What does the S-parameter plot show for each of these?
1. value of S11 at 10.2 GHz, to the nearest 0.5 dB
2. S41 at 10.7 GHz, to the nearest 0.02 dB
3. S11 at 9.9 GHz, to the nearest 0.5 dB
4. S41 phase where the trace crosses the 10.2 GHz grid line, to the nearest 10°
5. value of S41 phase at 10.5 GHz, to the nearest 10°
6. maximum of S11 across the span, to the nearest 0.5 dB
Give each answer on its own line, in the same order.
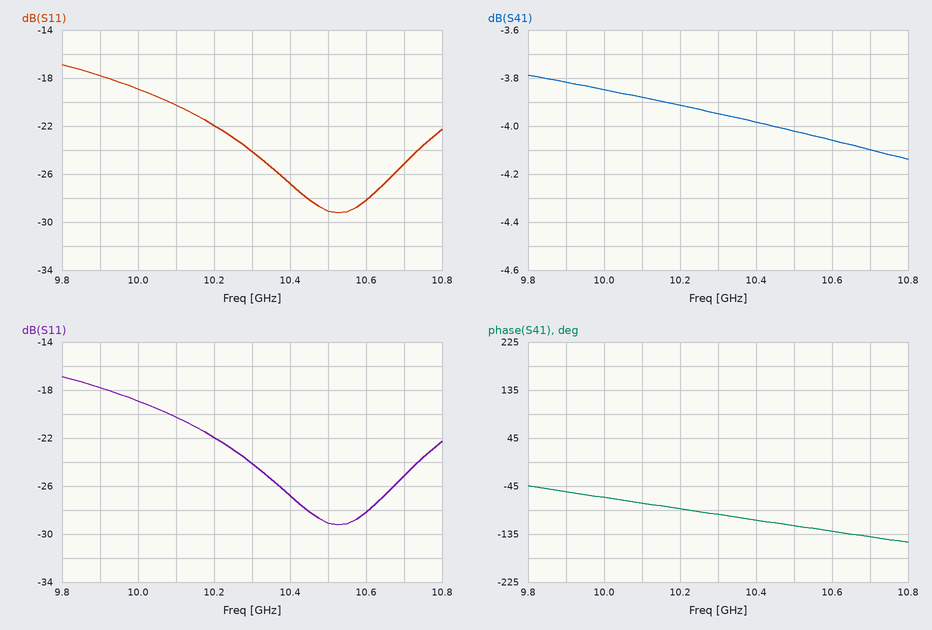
-22.0 dB
-4.10 dB
-18.0 dB
-90°
-120°
-17.0 dB
